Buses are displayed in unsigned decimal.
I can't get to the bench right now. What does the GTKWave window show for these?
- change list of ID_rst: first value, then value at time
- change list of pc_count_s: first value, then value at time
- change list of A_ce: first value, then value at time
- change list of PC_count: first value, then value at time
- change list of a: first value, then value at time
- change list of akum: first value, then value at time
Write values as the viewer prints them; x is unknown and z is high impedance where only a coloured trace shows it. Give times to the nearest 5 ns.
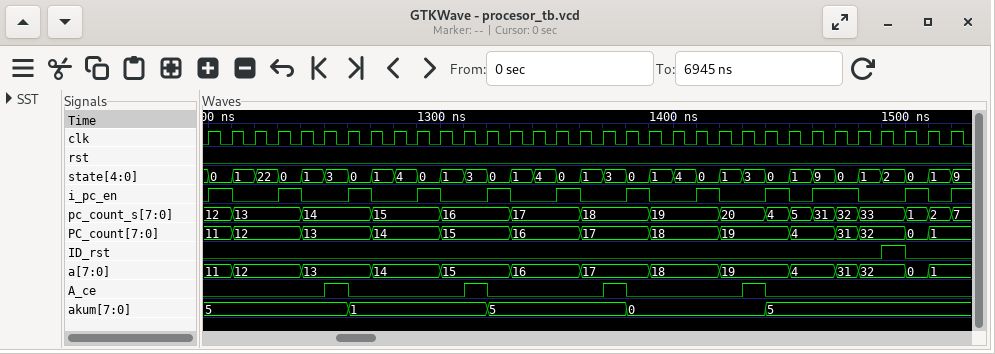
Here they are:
0, 1 at 1490 ns, 0 at 1500 ns
12, 13 at 1210 ns, 14 at 1240 ns, 15 at 1270 ns, 16 at 1300 ns, 17 at 1330 ns, 18 at 1360 ns, 19 at 1390 ns, 20 at 1420 ns, 4 at 1440 ns, 5 at 1450 ns, 31 at 1460 ns, 32 at 1470 ns, 33 at 1480 ns, 1 at 1500 ns, 2 at 1510 ns, 7 at 1520 ns
0, 1 at 1250 ns, 0 at 1260 ns, 1 at 1310 ns, 0 at 1320 ns, 1 at 1370 ns, 0 at 1380 ns, 1 at 1430 ns, 0 at 1440 ns
11, 12 at 1210 ns, 13 at 1240 ns, 14 at 1270 ns, 15 at 1300 ns, 16 at 1330 ns, 17 at 1360 ns, 18 at 1390 ns, 19 at 1420 ns, 4 at 1450 ns, 31 at 1470 ns, 32 at 1480 ns, 0 at 1500 ns, 1 at 1510 ns
11, 12 at 1210 ns, 13 at 1240 ns, 14 at 1270 ns, 15 at 1300 ns, 16 at 1330 ns, 17 at 1360 ns, 18 at 1390 ns, 19 at 1420 ns, 4 at 1450 ns, 31 at 1470 ns, 32 at 1480 ns, 0 at 1500 ns, 1 at 1510 ns
5, 1 at 1260 ns, 5 at 1320 ns, 0 at 1380 ns, 5 at 1440 ns
